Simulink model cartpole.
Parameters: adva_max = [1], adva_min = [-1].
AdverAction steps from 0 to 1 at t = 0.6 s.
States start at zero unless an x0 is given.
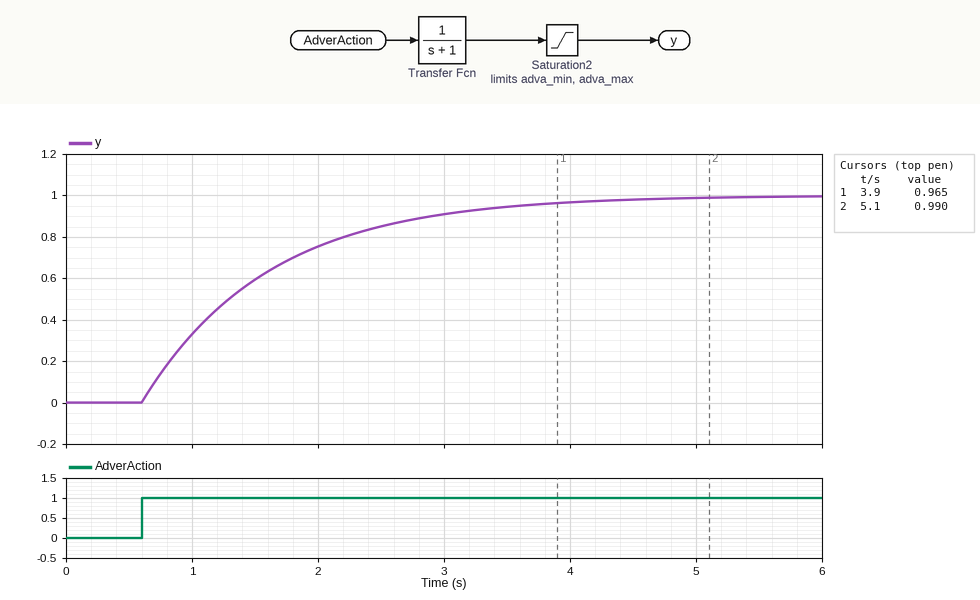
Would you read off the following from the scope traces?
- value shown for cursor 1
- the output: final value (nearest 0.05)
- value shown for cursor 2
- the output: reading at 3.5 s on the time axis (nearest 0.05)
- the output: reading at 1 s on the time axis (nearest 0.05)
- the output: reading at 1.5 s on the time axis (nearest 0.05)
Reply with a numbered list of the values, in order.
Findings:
1. 0.965
2. 1.00
3. 0.990
4. 0.95
5. 0.35
6. 0.60
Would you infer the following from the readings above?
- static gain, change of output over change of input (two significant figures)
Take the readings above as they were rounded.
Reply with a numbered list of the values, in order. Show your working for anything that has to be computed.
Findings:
1. (1 - 0) / (1 - 0) = 1.0
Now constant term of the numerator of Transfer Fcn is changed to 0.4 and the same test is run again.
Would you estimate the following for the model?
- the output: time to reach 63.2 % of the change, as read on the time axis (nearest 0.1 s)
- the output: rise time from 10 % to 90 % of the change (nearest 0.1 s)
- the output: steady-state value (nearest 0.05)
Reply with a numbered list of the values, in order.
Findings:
1. 1.6 s
2. 2.2 s
3. 0.40
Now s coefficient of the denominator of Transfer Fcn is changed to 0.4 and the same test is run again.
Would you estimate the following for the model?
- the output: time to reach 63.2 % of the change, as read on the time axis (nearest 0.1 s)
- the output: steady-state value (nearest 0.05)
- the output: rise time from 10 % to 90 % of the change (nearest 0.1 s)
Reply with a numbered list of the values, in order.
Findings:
1. 1.0 s
2. 1.00
3. 0.9 s
